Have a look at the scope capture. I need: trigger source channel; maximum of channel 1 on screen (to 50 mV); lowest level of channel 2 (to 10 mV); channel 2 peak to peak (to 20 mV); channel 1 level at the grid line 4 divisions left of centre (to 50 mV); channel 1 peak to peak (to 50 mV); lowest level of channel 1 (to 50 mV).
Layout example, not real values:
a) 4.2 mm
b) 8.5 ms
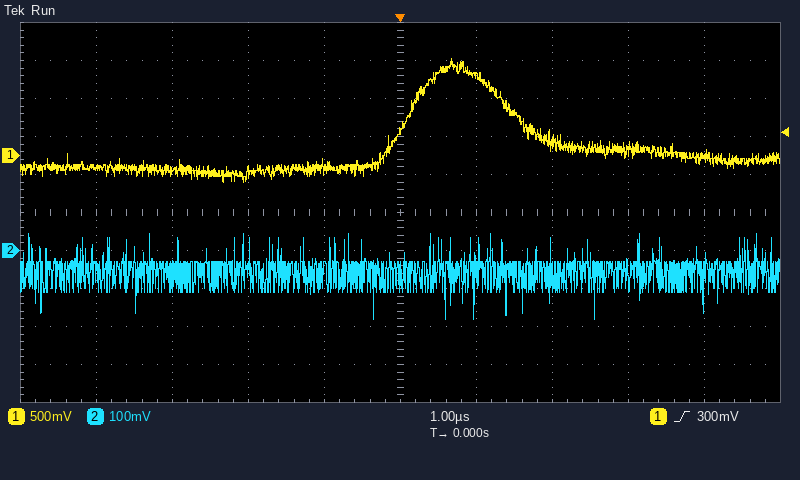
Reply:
a) channel 1
b) 1.30 V
c) -180 mV
d) 220 mV
e) -150 mV
f) 1.65 V
g) -350 mV
